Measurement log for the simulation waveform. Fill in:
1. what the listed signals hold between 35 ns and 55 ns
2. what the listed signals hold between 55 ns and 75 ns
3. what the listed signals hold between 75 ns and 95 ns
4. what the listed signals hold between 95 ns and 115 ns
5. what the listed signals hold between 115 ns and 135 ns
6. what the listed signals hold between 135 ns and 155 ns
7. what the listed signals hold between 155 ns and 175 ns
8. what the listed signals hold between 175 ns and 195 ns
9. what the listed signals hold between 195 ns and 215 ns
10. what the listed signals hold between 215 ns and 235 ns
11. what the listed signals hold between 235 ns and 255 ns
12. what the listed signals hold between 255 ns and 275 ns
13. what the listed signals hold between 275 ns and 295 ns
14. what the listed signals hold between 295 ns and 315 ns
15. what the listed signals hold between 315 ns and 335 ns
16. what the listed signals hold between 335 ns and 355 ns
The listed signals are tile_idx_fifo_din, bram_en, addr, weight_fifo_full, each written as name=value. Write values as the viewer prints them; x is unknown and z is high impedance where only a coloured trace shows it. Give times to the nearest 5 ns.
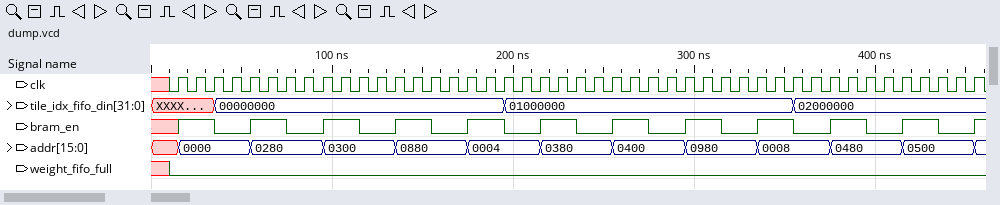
tile_idx_fifo_din=00000000, bram_en=0, addr=0000, weight_fifo_full=0
tile_idx_fifo_din=00000000, bram_en=1, addr=0280, weight_fifo_full=0
tile_idx_fifo_din=00000000, bram_en=0, addr=0280, weight_fifo_full=0
tile_idx_fifo_din=00000000, bram_en=1, addr=0300, weight_fifo_full=0
tile_idx_fifo_din=00000000, bram_en=0, addr=0300, weight_fifo_full=0
tile_idx_fifo_din=00000000, bram_en=1, addr=0880, weight_fifo_full=0
tile_idx_fifo_din=00000000, bram_en=0, addr=0880, weight_fifo_full=0
tile_idx_fifo_din=00000000, bram_en=1, addr=0004, weight_fifo_full=0
tile_idx_fifo_din=01000000, bram_en=0, addr=0004, weight_fifo_full=0
tile_idx_fifo_din=01000000, bram_en=1, addr=0380, weight_fifo_full=0
tile_idx_fifo_din=01000000, bram_en=0, addr=0380, weight_fifo_full=0
tile_idx_fifo_din=01000000, bram_en=1, addr=0400, weight_fifo_full=0
tile_idx_fifo_din=01000000, bram_en=0, addr=0400, weight_fifo_full=0
tile_idx_fifo_din=01000000, bram_en=1, addr=0980, weight_fifo_full=0
tile_idx_fifo_din=01000000, bram_en=0, addr=0980, weight_fifo_full=0
tile_idx_fifo_din=01000000, bram_en=1, addr=0008, weight_fifo_full=0
